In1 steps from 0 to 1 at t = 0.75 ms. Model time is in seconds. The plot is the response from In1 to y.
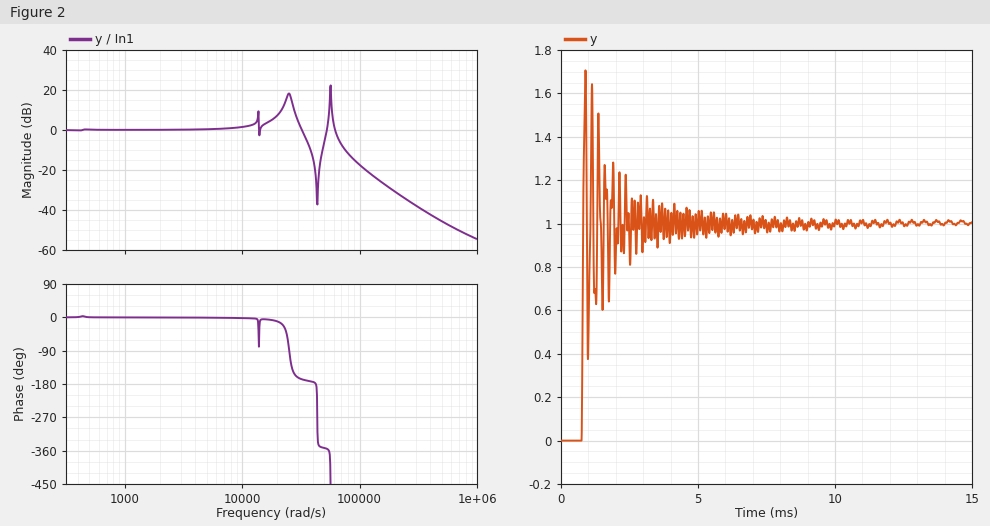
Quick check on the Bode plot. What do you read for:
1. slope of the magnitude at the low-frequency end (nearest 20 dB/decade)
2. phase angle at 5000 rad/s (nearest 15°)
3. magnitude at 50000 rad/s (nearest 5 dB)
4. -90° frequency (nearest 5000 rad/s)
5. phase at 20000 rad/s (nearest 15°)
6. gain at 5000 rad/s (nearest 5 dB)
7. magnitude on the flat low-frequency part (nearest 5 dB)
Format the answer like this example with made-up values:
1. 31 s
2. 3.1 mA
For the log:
1. 0 dB/decade
2. 0°
3. -5 dB
4. 25000 rad/s
5. -15°
6. 0 dB
7. 0 dB
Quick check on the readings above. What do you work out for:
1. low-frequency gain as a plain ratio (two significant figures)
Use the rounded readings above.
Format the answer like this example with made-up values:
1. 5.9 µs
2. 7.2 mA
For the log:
1. 1.0
